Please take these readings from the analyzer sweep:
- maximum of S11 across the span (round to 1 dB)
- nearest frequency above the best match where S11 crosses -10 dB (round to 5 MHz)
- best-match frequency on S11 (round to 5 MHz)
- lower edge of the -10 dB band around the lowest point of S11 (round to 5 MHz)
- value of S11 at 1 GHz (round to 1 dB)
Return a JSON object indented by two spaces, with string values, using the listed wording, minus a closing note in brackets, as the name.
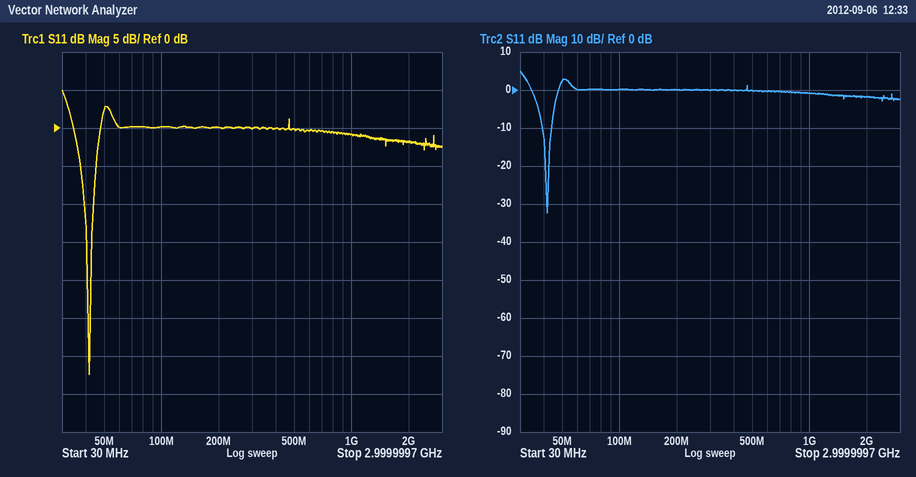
{
  "maximum of S11 across the span": "5 dB",
  "nearest frequency above the best match where S11 crosses -10 dB": "45 MHz",
  "best-match frequency on S11": "40 MHz",
  "lower edge of the -10 dB band around the lowest point of S11": "40 MHz",
  "value of S11 at 1 GHz": "-1 dB"
}
